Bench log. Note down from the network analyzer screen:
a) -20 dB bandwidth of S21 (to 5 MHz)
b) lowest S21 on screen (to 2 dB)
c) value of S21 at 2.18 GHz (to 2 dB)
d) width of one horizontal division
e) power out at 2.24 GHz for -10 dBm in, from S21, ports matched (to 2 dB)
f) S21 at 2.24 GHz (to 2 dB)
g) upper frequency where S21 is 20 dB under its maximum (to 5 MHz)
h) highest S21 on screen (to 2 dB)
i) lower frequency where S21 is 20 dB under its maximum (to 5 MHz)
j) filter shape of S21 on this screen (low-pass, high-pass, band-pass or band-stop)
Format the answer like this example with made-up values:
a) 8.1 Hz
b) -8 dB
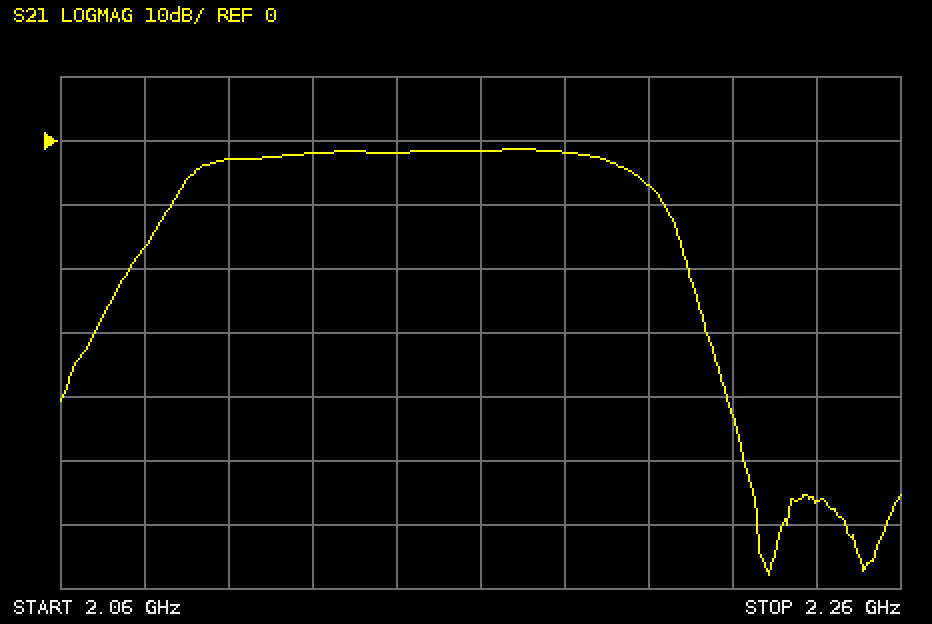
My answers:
a) 135 MHz
b) -68 dB
c) -2 dB
d) 20 MHz
e) -66 dBm
f) -56 dB
g) 2.210 GHz
h) -2 dB
i) 2.075 GHz
j) band-pass
